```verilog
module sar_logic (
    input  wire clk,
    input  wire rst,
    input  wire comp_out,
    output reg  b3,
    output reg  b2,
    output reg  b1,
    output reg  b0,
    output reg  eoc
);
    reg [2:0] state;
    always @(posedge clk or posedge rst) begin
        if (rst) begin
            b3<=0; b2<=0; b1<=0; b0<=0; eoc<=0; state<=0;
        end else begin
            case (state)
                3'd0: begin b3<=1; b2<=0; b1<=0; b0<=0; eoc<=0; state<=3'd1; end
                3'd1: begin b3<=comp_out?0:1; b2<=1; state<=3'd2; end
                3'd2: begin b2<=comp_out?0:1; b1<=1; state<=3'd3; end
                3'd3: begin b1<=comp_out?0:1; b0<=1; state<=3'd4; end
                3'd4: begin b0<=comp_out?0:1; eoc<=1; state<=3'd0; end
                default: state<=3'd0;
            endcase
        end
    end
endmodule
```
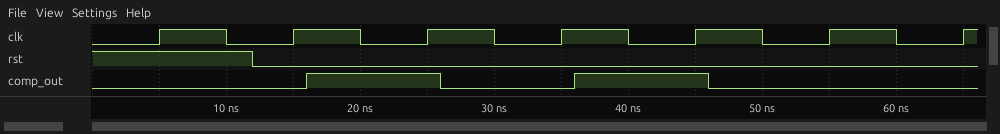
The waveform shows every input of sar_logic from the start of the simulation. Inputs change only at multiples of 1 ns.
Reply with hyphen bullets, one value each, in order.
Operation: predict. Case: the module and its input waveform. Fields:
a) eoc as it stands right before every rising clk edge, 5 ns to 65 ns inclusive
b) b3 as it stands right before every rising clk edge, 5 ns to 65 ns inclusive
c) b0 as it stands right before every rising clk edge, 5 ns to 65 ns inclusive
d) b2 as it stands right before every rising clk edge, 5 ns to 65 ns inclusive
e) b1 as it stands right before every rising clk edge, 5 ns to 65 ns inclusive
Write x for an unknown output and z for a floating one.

- 0 0 0 0 0 0 1
- 0 0 1 0 0 0 0
- 0 0 0 0 0 1 1
- 0 0 0 1 1 1 1
- 0 0 0 0 1 0 0
